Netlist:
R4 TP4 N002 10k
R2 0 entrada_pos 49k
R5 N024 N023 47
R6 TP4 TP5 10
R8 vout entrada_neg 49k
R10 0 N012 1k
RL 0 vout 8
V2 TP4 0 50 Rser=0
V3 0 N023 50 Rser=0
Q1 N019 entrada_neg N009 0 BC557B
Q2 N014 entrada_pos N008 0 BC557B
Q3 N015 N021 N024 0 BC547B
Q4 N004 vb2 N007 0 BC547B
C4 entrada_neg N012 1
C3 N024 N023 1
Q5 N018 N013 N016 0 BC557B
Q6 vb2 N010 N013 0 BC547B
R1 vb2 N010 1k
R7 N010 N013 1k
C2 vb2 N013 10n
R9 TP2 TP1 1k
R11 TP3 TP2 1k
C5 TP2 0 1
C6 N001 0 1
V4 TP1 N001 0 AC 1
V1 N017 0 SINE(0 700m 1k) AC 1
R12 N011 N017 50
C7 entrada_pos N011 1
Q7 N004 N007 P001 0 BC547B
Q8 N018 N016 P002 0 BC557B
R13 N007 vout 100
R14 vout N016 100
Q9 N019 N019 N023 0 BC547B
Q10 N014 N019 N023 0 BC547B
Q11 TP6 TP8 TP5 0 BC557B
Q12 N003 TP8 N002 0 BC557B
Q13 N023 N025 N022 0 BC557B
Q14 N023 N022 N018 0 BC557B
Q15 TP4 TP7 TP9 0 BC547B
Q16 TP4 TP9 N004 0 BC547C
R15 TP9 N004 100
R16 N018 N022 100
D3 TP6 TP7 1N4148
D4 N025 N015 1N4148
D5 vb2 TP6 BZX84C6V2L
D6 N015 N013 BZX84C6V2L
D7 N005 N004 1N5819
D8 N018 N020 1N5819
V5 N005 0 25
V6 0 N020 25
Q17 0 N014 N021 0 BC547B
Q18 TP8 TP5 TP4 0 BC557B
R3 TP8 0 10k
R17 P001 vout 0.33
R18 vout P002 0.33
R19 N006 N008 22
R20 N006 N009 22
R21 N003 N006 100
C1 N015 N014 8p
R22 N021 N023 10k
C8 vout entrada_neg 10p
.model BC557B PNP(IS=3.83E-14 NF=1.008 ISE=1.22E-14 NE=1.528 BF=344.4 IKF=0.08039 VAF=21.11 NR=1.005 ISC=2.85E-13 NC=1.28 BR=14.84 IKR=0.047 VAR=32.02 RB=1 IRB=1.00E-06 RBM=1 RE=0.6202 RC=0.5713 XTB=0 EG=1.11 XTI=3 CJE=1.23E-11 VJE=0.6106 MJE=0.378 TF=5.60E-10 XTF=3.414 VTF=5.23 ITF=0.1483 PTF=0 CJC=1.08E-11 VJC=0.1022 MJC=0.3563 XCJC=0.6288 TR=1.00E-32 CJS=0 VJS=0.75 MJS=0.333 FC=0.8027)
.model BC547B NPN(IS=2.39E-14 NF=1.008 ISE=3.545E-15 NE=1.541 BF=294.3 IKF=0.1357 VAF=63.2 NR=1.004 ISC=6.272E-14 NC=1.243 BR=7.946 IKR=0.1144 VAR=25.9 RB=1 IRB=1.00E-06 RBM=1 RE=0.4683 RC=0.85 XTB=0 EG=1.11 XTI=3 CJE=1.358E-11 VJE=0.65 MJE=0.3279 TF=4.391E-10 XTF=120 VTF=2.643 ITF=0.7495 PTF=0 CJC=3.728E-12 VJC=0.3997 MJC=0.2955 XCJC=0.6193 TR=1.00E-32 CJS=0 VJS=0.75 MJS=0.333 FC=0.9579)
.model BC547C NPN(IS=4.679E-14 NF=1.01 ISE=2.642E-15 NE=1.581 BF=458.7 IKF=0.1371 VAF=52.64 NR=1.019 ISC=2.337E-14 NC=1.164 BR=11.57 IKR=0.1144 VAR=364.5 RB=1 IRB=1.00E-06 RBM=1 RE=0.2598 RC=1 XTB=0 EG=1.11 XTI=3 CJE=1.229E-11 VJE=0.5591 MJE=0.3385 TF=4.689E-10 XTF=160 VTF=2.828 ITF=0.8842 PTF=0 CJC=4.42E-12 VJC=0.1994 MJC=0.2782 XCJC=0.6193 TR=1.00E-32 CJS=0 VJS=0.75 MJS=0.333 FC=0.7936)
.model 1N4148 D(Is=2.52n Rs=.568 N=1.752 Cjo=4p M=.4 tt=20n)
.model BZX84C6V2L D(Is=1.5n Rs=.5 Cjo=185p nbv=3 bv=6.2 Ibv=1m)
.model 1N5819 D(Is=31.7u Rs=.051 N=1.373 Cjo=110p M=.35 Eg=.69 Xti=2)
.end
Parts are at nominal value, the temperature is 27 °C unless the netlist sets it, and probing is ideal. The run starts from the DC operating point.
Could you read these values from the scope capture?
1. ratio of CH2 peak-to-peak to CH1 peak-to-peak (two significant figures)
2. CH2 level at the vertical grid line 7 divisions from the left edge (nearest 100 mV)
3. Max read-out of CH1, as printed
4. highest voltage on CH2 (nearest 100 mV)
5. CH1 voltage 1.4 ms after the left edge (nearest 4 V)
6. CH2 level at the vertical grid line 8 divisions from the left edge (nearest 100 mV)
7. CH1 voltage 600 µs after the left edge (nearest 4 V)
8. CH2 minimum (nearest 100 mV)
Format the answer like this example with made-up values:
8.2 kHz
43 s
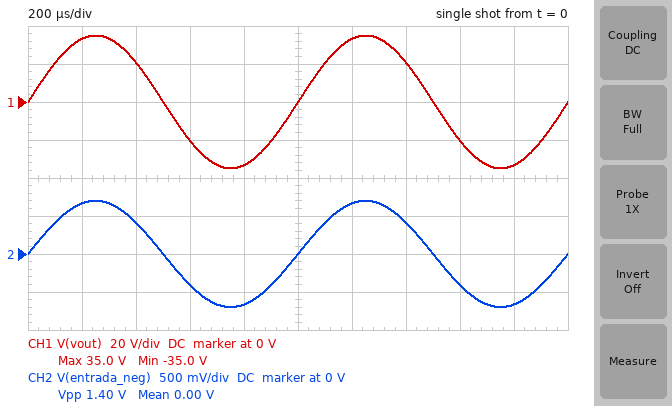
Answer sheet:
0.020
400 mV
35.0 V
700 mV
20 V
-400 mV
-20 V
-700 mV
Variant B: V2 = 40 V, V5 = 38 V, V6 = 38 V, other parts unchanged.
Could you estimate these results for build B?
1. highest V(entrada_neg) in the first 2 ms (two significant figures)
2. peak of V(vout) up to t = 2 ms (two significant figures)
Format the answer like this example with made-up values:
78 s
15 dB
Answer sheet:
570 mV
29 V
